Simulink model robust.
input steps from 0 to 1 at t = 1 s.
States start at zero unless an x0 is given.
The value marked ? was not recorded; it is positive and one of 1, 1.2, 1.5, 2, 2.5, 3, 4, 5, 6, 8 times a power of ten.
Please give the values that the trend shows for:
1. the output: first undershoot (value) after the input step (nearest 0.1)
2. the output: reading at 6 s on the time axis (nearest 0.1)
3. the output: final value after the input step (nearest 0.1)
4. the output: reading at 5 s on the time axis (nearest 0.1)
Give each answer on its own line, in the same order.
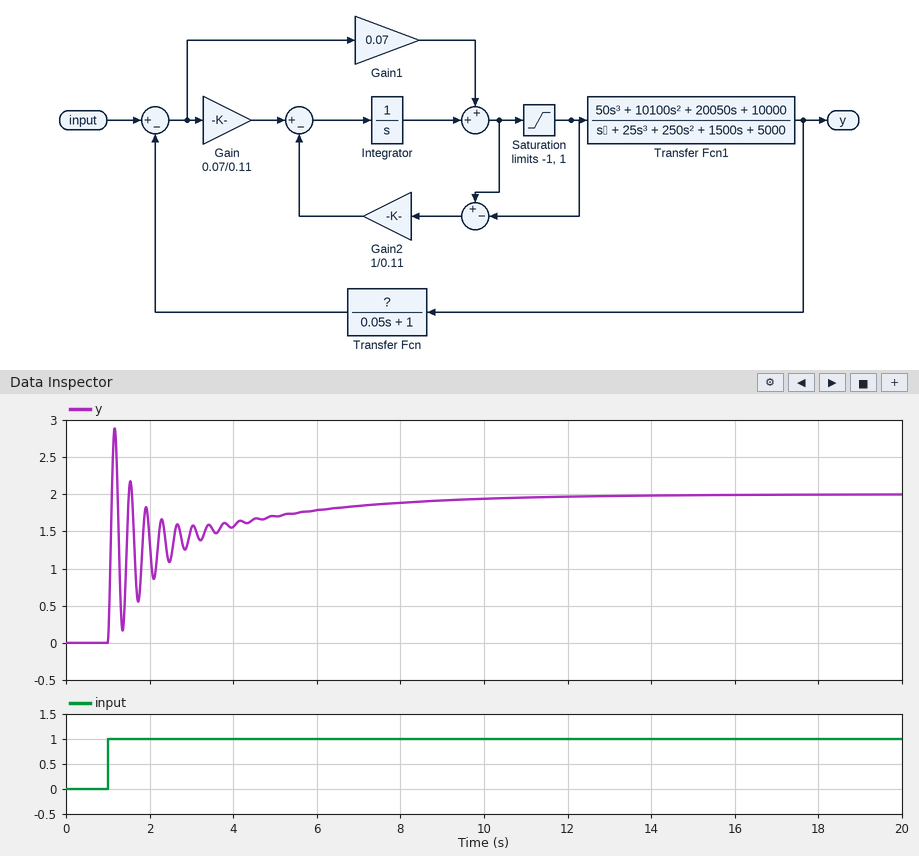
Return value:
0.2
1.8
2.0
1.7
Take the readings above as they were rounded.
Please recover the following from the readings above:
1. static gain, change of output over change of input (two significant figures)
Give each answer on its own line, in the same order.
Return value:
2.0
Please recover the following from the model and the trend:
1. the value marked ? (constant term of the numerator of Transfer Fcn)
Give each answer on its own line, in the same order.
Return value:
0.5
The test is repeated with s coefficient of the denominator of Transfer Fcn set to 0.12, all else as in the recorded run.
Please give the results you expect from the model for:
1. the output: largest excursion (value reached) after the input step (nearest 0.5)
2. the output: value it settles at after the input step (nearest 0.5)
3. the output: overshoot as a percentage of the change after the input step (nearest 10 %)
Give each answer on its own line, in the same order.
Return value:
3.5
2.0
80 %
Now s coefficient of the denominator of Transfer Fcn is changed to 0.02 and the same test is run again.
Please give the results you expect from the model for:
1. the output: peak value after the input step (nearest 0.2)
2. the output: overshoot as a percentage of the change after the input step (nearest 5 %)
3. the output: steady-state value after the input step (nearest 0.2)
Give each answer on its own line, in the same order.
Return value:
2.4
20 %
2.0
